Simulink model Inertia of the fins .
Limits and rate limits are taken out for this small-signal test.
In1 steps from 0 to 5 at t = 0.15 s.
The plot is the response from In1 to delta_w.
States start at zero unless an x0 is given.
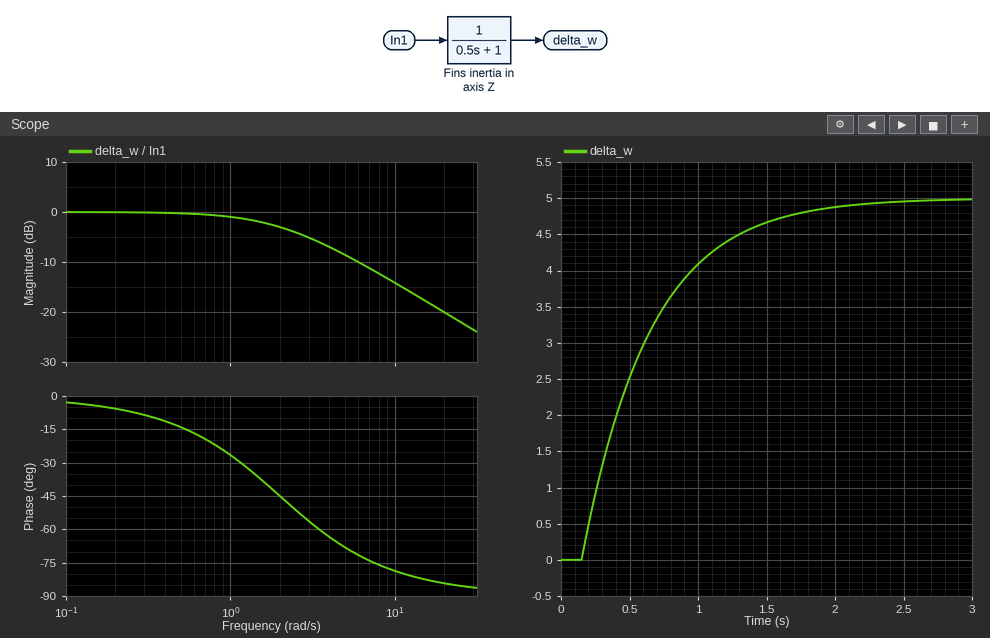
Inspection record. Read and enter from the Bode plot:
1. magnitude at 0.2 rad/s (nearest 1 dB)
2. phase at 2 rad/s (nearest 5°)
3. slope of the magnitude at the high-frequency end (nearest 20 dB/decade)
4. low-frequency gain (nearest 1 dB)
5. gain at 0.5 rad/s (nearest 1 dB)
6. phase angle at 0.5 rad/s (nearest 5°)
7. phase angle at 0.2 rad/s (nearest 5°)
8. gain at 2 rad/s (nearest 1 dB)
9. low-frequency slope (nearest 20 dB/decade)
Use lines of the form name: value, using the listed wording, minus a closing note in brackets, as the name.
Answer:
magnitude at 0.2 rad/s: 0 dB
phase at 2 rad/s: -45°
slope of the magnitude at the high-frequency end: -20 dB/decade
low-frequency gain: 0 dB
gain at 0.5 rad/s: 0 dB
phase angle at 0.5 rad/s: -15°
phase angle at 0.2 rad/s: -5°
gain at 2 rad/s: -3 dB
low-frequency slope: 0 dB/decade
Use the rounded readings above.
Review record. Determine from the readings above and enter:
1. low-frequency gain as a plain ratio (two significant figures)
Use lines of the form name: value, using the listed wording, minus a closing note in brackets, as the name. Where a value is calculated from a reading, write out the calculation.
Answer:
low-frequency gain as a plain ratio: 10^(0 / 20) = 1.0
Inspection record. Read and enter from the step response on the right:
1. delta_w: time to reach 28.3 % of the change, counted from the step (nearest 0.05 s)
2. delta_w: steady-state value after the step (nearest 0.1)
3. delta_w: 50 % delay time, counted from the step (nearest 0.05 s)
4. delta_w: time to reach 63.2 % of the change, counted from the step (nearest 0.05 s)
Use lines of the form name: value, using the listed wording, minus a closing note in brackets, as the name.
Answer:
delta_w: time to reach 28.3 % of the change, counted from the step: 0.15 s
delta_w: steady-state value after the step: 5.0
delta_w: 50 % delay time, counted from the step: 0.35 s
delta_w: time to reach 63.2 % of the change, counted from the step: 0.50 s
